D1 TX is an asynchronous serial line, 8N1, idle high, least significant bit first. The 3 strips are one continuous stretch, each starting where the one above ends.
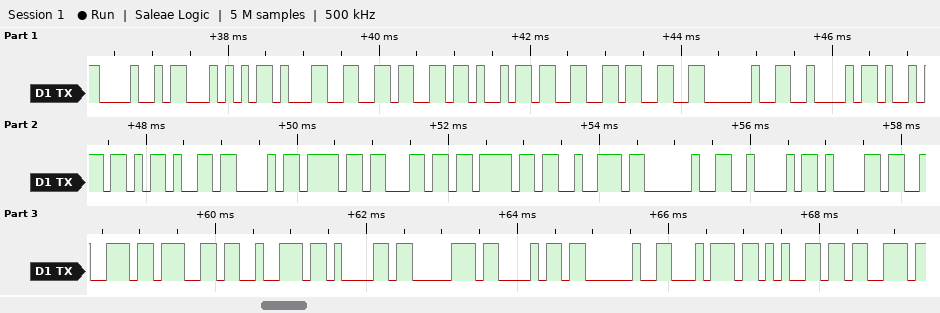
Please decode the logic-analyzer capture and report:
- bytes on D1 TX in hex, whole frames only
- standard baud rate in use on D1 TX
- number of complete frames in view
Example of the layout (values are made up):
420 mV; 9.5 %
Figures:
48 54 31 36 4B 33 33 20 42 69 2D 43 6F 6C 6F 72 20 42 61 72 67 72 61 70 68 20 74 65 73; 9600 baud; 29
